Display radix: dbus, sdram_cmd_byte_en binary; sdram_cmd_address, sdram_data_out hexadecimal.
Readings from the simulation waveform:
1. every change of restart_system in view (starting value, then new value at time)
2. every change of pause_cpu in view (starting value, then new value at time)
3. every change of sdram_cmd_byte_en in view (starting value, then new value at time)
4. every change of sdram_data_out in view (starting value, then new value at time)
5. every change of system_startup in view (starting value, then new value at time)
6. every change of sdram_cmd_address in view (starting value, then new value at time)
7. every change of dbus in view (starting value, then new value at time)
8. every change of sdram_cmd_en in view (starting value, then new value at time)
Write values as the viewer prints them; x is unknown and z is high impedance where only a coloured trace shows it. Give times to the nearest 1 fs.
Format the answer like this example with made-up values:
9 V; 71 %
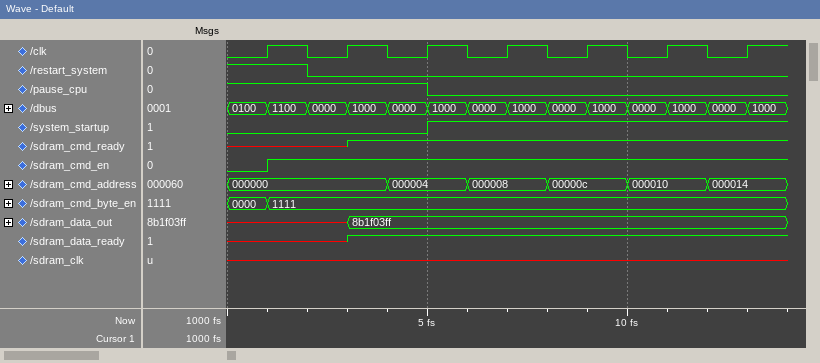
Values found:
1, 0 at 2 fs; 1, 0 at 5 fs; 0000, 1111 at 1 fs; x, 8b1f03ff at 3 fs; 0, 1 at 5 fs; 000000, 000004 at 4 fs, 000008 at 6 fs, 00000c at 8 fs, 000010 at 10 fs, 000014 at 12 fs; 0100, 1100 at 1 fs, 0000 at 2 fs, 1000 at 3 fs, 0000 at 4 fs, 1000 at 5 fs, 0000 at 6 fs, 1000 at 7 fs, 0000 at 8 fs, 1000 at 9 fs, 0000 at 10 fs, 1000 at 11 fs, 0000 at 12 fs, 1000 at 13 fs; 0, 1 at 1 fs
